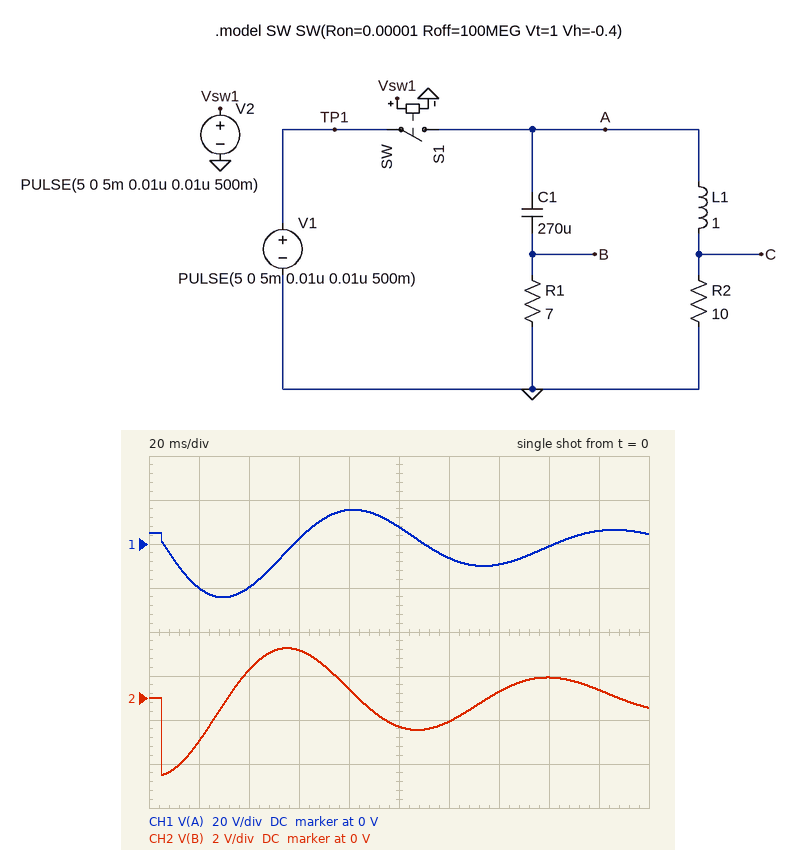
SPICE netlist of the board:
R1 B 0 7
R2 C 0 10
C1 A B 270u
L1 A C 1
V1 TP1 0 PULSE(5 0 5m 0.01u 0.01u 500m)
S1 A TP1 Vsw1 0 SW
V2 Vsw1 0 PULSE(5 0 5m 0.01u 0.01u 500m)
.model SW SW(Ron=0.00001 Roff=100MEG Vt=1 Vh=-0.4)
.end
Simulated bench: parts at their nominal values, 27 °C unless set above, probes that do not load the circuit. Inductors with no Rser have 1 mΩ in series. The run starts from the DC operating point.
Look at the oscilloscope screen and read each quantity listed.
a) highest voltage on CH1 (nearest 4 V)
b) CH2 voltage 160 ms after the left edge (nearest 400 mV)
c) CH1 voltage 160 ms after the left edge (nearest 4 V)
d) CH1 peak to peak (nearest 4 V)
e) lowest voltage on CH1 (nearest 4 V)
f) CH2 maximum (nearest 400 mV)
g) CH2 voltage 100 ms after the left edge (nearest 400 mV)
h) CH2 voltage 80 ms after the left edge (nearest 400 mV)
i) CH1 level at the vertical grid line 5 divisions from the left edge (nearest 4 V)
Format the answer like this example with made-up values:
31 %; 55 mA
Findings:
16 V; 800 mV; 0 V; 40 V; -24 V; 2.4 V; -1.2 V; 400 mV; 8 V
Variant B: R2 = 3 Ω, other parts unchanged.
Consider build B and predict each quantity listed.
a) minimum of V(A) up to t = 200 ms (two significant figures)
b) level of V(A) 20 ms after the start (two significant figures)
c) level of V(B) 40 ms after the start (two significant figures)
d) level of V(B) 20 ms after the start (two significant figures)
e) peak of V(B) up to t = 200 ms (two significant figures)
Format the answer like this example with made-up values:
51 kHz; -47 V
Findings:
-90 V; -78 V; 5.4 V; -6.4 V; 9.1 V
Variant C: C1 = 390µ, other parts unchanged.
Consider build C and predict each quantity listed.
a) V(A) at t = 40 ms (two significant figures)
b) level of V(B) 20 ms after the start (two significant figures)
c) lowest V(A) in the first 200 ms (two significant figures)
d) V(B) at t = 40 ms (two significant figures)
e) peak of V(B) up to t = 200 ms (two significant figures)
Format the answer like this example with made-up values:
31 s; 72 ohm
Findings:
-18 V; -2.3 V; -19 V; 380 mV; 2.1 V
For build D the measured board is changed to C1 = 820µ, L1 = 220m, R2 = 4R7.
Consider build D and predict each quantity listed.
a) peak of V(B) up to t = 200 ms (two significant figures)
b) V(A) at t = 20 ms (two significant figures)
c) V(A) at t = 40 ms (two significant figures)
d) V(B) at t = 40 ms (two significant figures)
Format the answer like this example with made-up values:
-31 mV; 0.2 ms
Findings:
2.5 V; -10 V; -3.4 V; 2.4 V
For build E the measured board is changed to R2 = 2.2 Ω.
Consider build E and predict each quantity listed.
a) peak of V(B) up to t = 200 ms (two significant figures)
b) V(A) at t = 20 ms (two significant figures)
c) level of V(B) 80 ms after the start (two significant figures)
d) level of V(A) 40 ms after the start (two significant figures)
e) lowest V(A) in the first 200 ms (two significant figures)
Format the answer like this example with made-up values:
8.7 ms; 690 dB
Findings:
13 V; -110 V; 1.4 V; -95 V; -120 V
